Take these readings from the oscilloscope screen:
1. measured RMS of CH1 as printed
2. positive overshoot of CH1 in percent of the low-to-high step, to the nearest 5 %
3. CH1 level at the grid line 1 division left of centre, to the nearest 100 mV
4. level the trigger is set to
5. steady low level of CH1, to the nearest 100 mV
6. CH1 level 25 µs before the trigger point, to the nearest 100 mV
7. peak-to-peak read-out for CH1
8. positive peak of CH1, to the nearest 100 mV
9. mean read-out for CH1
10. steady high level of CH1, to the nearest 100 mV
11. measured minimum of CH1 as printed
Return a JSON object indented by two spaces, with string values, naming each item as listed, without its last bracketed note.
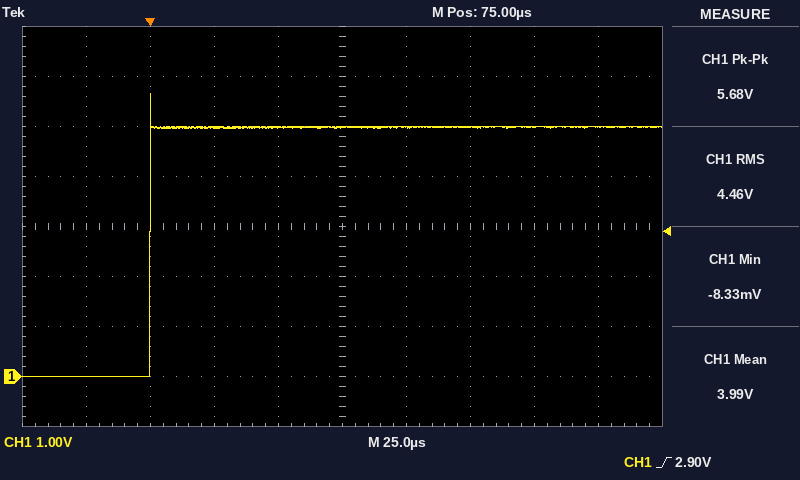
{
  "measured RMS of CH1 as printed": "4.46 V",
  "positive overshoot of CH1 in percent of the low-to-high step, to the nearest 5 %": "15 %",
  "CH1 level at the grid line 1 division left of centre, to the nearest 100 mV": "5.0 V",
  "level the trigger is set to": "2.90 V",
  "steady low level of CH1, to the nearest 100 mV": "0.0 V",
  "CH1 level 25 µs before the trigger point, to the nearest 100 mV": "0.0 V",
  "peak-to-peak read-out for CH1": "5.68 V",
  "positive peak of CH1, to the nearest 100 mV": "5.7 V",
  "mean read-out for CH1": "3.99 V",
  "steady high level of CH1, to the nearest 100 mV": "5.0 V",
  "measured minimum of CH1 as printed": "-8.33 mV"
}
